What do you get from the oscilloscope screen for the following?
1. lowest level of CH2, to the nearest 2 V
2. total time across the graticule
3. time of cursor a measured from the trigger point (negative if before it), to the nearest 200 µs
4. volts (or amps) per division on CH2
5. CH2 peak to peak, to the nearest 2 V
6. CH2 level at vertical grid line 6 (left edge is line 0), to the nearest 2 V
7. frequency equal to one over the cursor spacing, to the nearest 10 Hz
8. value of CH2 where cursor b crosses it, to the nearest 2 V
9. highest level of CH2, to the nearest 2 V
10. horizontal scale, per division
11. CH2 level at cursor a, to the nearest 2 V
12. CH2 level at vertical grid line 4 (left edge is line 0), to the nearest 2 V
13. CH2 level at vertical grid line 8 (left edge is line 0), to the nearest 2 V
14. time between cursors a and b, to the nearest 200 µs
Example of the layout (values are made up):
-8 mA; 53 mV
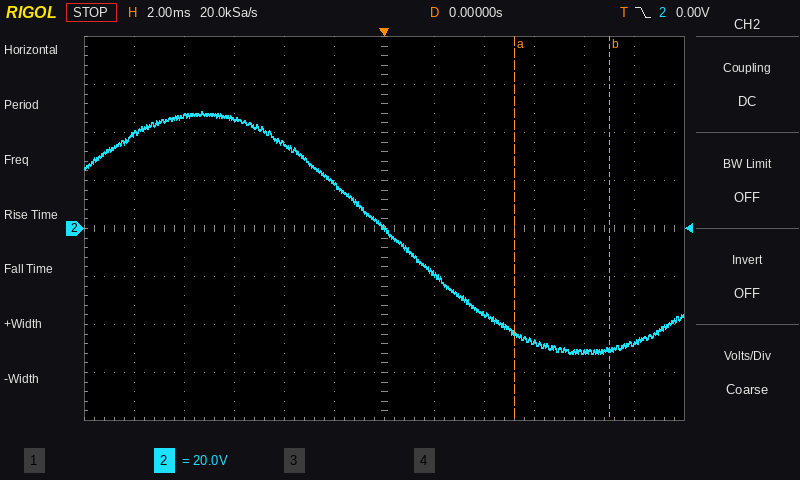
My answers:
-52 V; 24 ms; +5.2 ms; 20 V; 100 V; 0 V; 260 Hz; -50 V; 48 V; 2 ms; -44 V; 36 V; -36 V; 3.8 ms
